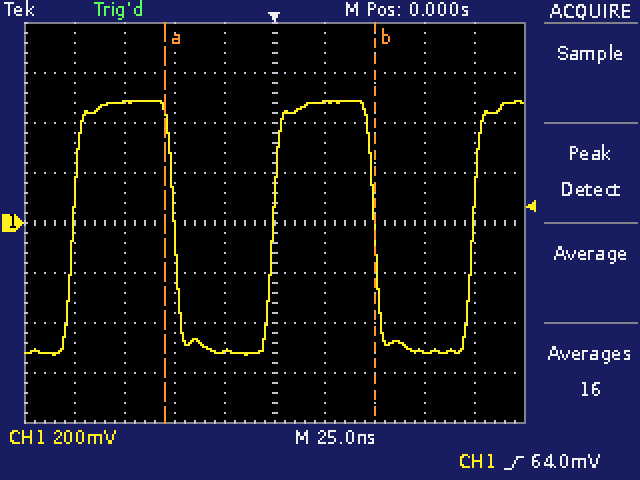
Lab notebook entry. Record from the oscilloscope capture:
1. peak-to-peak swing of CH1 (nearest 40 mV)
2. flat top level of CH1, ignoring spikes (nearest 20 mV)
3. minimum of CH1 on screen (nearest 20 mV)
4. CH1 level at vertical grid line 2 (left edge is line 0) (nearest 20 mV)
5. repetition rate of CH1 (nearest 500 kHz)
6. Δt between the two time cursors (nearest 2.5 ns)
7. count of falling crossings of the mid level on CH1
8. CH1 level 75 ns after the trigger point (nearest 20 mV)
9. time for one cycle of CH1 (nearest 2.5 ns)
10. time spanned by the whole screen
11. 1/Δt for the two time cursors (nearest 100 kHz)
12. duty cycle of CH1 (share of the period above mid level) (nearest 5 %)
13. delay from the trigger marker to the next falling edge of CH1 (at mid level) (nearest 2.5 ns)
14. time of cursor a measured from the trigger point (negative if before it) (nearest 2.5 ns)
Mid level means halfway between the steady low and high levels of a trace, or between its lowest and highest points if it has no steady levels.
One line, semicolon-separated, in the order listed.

1.00 V; 480 mV; -520 mV; 480 mV; 10.0 MHz; 105.0 ns; 2; -520 mV; 100.0 ns; 250 ns; 9.5 MHz; 50 %; 50.0 ns; -55.0 ns
